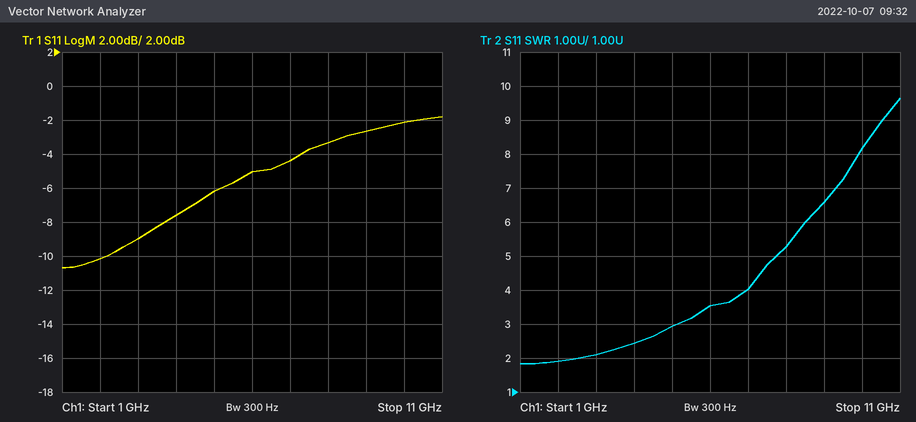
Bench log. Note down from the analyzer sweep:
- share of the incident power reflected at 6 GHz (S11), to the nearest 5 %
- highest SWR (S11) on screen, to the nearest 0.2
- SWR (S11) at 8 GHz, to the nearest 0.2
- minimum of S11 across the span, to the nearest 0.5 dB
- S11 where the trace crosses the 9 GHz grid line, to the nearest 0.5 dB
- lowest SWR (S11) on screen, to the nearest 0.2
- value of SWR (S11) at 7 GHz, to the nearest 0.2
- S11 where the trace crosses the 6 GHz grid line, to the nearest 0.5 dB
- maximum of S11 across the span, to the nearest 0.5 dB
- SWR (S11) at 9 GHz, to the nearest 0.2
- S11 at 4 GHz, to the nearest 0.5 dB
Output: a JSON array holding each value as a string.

["30 %", "9.6", "5.2", "-10.5 dB", "-2.5 dB", "1.8", "4.0", "-5.0 dB", "-2.0 dB", "6.6", "-7.5 dB"]
